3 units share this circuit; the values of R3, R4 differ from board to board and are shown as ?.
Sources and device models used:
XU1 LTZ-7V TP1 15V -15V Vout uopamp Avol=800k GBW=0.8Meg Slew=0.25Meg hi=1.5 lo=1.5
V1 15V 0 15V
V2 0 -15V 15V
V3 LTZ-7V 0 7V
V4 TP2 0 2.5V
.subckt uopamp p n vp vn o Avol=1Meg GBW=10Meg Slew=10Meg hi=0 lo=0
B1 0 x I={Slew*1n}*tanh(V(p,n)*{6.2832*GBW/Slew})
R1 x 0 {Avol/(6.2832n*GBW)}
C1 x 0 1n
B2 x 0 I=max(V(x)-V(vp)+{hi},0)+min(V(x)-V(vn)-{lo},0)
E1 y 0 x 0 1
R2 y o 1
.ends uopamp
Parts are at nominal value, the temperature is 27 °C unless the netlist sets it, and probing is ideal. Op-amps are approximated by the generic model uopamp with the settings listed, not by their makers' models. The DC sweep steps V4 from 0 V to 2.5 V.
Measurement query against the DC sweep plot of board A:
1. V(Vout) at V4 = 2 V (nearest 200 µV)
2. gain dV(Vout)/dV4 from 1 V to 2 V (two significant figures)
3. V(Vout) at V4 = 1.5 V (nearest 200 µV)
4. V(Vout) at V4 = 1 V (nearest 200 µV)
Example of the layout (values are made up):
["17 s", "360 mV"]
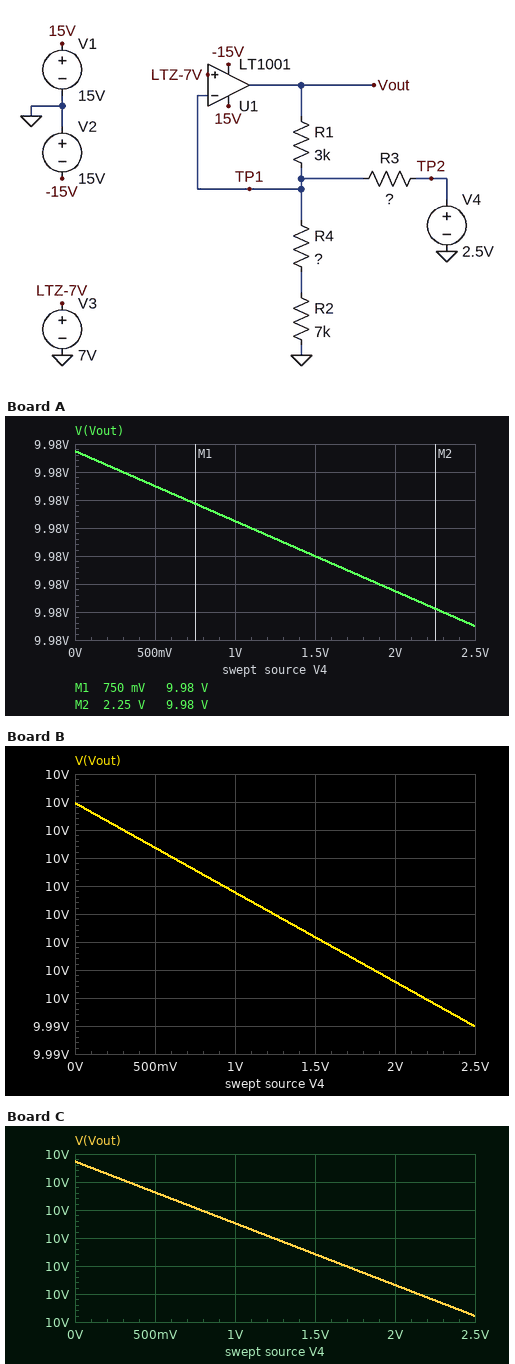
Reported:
["9.9778 V", "-0.0025 V/V", "9.9790 V", "9.9802 V"]
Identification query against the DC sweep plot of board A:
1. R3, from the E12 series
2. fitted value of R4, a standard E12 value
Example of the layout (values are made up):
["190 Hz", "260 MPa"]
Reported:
["1.2 MΩ", "82 Ω"]
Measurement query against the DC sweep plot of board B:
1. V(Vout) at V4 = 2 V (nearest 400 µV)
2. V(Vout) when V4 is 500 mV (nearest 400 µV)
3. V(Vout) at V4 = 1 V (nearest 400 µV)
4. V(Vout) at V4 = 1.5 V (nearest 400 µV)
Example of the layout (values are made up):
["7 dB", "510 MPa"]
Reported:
["9.9972 V", "10.0068 V", "10.0036 V", "10.0004 V"]
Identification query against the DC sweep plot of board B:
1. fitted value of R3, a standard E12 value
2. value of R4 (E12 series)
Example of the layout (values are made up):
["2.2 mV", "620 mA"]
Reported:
["470 kΩ", "82 Ω"]
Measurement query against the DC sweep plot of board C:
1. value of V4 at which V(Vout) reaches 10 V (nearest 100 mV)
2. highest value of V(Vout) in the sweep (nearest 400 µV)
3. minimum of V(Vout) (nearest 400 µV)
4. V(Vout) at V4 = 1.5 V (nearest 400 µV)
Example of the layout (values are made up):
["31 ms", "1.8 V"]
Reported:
["800 mV", "10.0216 V", "10.0104 V", "10.0148 V"]
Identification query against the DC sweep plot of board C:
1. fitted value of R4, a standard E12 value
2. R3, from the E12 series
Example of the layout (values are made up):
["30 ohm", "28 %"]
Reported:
["22 Ω", "680 kΩ"]
